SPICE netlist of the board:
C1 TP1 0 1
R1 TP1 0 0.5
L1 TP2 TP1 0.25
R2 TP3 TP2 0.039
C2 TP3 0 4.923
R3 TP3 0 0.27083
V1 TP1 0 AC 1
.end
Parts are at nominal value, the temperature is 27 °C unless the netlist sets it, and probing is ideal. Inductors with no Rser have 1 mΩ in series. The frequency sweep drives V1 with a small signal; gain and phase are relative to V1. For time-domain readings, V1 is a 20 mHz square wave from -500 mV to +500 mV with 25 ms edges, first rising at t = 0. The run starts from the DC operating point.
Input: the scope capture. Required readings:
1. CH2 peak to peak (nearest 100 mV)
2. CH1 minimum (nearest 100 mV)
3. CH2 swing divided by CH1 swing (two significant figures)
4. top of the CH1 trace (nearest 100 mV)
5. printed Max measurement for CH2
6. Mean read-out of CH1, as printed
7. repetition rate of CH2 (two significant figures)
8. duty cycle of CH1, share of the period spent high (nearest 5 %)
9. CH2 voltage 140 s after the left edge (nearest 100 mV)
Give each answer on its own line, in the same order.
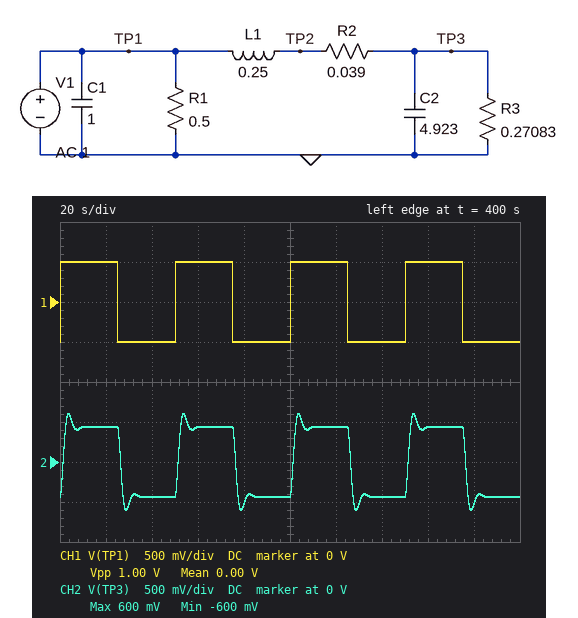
1.2 V
-500 mV
1.2
500 mV
600 mV
0.00 V
20 mHz
50 %
-400 mV
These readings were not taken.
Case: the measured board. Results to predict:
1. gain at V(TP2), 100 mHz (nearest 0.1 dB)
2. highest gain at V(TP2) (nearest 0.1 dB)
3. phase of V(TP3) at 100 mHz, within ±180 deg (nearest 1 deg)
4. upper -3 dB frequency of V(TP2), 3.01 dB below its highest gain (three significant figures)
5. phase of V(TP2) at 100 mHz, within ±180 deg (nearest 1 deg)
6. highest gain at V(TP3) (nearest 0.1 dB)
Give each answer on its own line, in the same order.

1.5 dB
1.6 dB
-47 deg
182 mHz
-41 deg
0.4 dB
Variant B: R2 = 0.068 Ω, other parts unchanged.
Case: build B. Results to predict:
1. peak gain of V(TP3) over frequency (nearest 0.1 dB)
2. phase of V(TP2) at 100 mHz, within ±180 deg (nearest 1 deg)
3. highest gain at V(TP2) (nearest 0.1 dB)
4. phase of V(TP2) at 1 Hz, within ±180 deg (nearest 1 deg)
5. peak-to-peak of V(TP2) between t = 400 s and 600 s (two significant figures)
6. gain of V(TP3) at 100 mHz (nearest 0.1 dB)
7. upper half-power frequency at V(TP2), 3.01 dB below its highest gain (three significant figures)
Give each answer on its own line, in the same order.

-0.8 dB
-36 deg
1.3 dB
-111 deg
1.3 V
-0.9 dB
191 mHz
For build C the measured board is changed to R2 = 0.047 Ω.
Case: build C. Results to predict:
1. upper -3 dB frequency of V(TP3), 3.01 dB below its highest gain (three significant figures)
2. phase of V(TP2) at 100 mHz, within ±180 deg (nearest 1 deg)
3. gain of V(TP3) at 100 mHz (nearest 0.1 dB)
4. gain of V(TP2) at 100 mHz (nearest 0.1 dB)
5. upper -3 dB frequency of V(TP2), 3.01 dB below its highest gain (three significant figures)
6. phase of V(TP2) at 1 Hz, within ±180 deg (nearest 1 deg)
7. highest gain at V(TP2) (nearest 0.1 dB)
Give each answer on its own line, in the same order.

183 mHz
-39 deg
0 dB
1.4 dB
185 mHz
-120 deg
1.5 dB
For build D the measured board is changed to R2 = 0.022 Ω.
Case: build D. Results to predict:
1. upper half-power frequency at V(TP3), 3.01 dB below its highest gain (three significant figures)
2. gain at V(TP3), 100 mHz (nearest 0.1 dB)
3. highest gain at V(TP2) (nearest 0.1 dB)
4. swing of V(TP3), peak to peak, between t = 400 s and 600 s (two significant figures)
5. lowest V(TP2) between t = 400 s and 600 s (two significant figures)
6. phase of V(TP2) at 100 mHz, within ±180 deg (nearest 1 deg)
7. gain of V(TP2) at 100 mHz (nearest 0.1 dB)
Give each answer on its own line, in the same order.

177 mHz
1.1 dB
1.9 dB
1.3 V
-710 mV
-44 deg
1.8 dB
